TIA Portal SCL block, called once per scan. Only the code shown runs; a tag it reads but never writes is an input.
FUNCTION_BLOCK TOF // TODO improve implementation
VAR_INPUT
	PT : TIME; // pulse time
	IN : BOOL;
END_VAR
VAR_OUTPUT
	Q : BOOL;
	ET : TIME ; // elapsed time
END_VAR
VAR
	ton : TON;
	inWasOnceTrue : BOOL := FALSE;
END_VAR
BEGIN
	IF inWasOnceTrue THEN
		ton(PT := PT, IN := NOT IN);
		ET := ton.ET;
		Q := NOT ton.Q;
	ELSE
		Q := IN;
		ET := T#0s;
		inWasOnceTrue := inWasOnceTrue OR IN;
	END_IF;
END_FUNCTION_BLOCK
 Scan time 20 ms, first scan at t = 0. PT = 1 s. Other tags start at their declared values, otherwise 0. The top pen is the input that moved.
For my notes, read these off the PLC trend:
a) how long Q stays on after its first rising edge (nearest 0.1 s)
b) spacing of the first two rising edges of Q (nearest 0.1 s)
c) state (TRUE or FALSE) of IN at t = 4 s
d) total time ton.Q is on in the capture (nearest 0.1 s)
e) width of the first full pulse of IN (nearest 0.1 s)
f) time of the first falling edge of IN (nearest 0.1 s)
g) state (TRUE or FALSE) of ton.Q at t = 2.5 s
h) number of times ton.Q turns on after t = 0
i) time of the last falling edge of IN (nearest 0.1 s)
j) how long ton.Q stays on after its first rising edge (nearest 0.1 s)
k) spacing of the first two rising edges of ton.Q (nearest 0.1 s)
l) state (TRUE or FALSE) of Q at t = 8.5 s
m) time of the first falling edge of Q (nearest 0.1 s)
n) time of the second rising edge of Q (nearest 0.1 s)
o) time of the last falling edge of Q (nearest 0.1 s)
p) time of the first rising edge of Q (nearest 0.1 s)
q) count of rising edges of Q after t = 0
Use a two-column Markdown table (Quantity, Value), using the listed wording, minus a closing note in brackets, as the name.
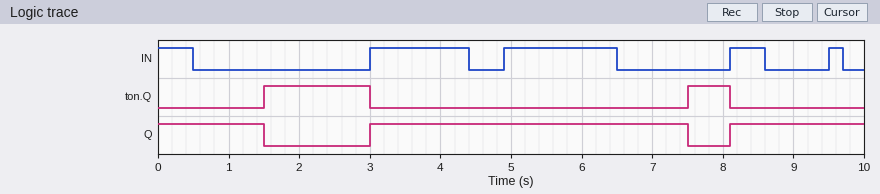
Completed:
| Quantity | Value |
|---|---|
| how long Q stays on after its first rising edge | 4.5 s |
| spacing of the first two rising edges of Q | 5.1 s |
| state (TRUE or FALSE) of IN at t = 4 s | TRUE |
| total time ton.Q is on in the capture | 2.1 s |
| width of the first full pulse of IN | 1.4 s |
| time of the first falling edge of IN | 0.5 s |
| state (TRUE or FALSE) of ton.Q at t = 2.5 s | TRUE |
| number of times ton.Q turns on after t = 0 | 2 |
| time of the last falling edge of IN | 9.7 s |
| how long ton.Q stays on after its first rising edge | 1.5 s |
| spacing of the first two rising edges of ton.Q | 6.0 s |
| state (TRUE or FALSE) of Q at t = 8.5 s | TRUE |
| time of the first falling edge of Q | 1.5 s |
| time of the second rising edge of Q | 8.1 s |
| time of the last falling edge of Q | 7.5 s |
| time of the first rising edge of Q | 3.0 s |
| count of rising edges of Q after t = 0 | 2 |
